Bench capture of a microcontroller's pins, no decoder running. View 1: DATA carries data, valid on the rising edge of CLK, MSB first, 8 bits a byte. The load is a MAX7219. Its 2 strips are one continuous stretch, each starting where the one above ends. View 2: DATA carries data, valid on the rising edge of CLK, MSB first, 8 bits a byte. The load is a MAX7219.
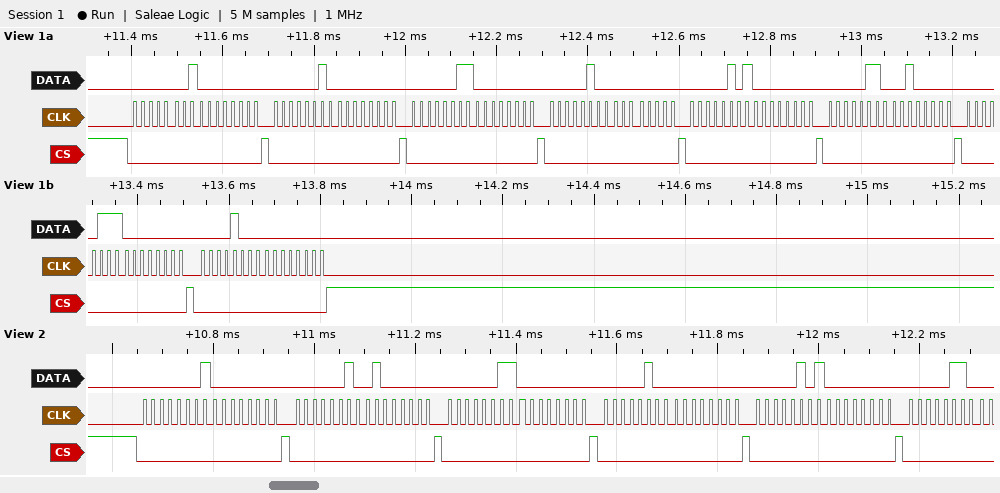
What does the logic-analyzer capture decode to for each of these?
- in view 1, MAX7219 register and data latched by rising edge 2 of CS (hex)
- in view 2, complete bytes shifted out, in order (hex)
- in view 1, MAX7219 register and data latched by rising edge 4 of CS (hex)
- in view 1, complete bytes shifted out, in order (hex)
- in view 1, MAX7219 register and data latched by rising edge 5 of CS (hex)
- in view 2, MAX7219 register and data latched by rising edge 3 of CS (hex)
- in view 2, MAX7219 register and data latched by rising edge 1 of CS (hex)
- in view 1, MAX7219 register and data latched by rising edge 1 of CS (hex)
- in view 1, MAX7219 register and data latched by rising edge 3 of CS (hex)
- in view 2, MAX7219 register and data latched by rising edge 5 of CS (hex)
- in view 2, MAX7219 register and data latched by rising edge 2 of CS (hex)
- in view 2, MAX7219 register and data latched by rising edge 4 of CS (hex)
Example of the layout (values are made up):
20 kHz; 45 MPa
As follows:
register 0x2, data 0x00; 0x01 0x00 0x02 0x40 0x03 0x00 0x04 0x00 0x05 0x00 0x06; register 0x4, data 0x00; 01 00 02 00 03 00 04 00 05 00 06 20 07 00 08 00; register 0x5, data 0x00; register 0x3, data 0x00; register 0x1, data 0x00; register 0x1, data 0x00; register 0x3, data 0x00; register 0x5, data 0x00; register 0x2, data 0x40; register 0x4, data 0x00
